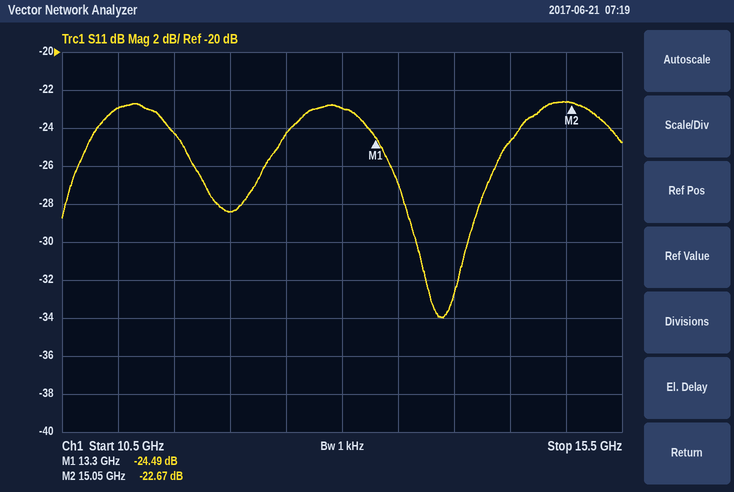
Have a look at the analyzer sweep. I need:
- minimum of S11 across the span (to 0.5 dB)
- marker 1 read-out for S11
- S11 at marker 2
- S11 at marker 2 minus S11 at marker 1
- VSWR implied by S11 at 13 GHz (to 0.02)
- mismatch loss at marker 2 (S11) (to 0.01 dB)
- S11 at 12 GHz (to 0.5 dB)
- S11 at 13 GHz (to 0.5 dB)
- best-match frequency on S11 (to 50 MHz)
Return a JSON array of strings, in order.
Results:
["-34.0 dB", "-24.49 dB", "-22.67 dB", "1.82 dB", "1.16", "0.02 dB", "-28.5 dB", "-23.0 dB", "13.90 GHz"]
